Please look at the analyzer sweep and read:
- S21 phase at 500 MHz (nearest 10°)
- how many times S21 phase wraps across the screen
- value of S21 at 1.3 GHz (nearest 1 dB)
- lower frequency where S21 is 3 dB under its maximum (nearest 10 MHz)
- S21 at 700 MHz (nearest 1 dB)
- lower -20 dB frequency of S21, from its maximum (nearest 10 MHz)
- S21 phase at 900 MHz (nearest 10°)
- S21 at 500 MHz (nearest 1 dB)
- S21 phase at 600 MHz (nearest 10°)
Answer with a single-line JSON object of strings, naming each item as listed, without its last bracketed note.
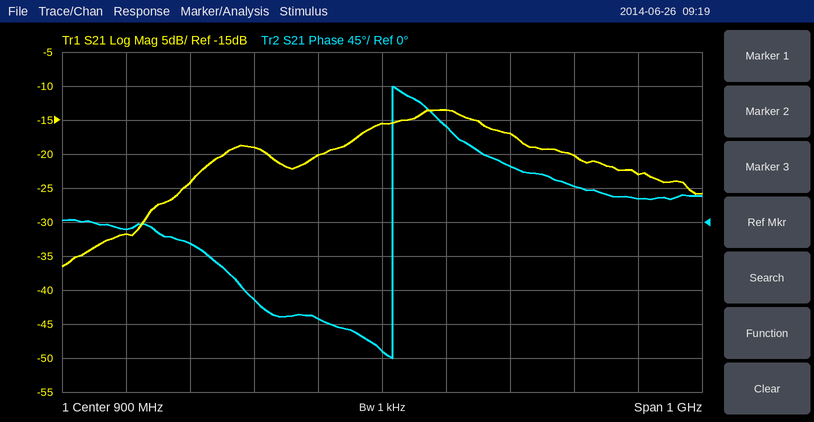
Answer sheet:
{"S21 phase at 500 MHz": "-10°", "how many times S21 phase wraps across the screen": "1", "value of S21 at 1.3 GHz": "-23 dB", "lower frequency where S21 is 3 dB under its maximum": "880 MHz", "S21 at 700 MHz": "-19 dB", "lower -20 dB frequency of S21, from its maximum": "450 MHz", "S21 phase at 900 MHz": "-170°", "S21 at 500 MHz": "-32 dB", "S21 phase at 600 MHz": "-30°"}
